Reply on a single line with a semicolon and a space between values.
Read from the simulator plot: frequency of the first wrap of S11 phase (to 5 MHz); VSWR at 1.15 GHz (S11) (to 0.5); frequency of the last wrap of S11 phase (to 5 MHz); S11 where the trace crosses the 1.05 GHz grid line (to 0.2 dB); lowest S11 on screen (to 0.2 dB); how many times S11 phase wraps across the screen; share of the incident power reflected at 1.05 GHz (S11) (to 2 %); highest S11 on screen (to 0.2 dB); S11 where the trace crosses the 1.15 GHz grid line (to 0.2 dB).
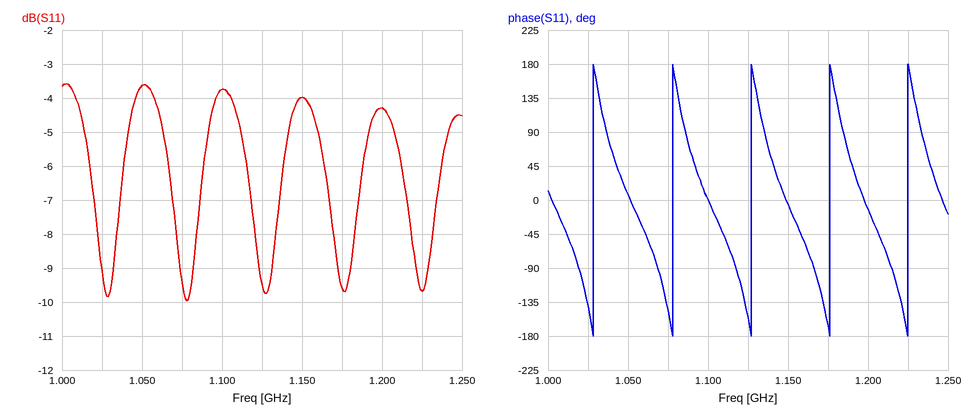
1.030 GHz; 4.5; 1.225 GHz; -3.6 dB; -10.0 dB; 5; 44 %; -3.6 dB; -4.0 dB
